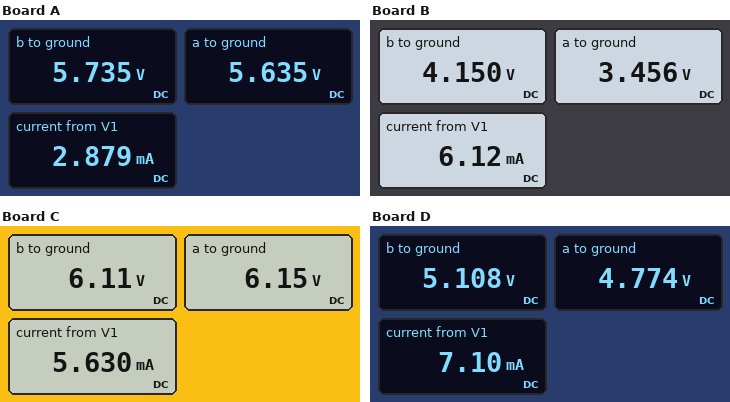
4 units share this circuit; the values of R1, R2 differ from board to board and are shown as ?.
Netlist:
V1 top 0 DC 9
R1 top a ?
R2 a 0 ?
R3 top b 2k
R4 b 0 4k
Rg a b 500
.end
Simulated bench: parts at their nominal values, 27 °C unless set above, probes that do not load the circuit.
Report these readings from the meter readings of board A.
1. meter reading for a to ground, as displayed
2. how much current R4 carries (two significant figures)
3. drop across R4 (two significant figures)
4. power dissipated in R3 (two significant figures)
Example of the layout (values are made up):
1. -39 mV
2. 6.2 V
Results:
1. 5.635 V
2. 1.4 mA
3. 5.7 V
4. 5.3 mW
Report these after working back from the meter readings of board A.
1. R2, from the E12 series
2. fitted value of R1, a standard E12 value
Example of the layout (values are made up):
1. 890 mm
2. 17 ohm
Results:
1. 3.9 kΩ
2. 2.7 kΩ
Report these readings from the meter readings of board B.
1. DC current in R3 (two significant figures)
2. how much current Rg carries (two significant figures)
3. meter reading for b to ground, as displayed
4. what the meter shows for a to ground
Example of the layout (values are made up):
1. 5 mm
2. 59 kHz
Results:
1. 2.4 mA
2. 1.4 mA
3. 4.150 V
4. 3.456 V
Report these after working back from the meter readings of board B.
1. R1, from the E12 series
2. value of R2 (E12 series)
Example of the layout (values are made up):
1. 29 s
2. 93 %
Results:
1. 1.5 kΩ
2. 680 Ω
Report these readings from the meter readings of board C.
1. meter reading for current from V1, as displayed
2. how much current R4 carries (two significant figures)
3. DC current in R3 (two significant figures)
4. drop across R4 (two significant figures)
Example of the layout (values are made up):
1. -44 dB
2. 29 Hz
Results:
1. 5.630 mA
2. 1.5 mA
3. 1.4 mA
4. 6.1 V
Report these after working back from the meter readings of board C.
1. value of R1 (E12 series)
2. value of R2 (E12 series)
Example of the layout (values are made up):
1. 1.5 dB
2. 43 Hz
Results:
1. 680 Ω
2. 1.5 kΩ
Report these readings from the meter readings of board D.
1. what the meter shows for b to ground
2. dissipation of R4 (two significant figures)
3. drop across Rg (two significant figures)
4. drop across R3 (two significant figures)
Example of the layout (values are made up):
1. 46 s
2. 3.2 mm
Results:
1. 5.108 V
2. 6.5 mW
3. 330 mV
4. 3.9 V
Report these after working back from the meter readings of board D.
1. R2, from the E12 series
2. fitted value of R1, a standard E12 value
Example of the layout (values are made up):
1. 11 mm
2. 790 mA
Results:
1. 820 Ω
2. 820 Ω
